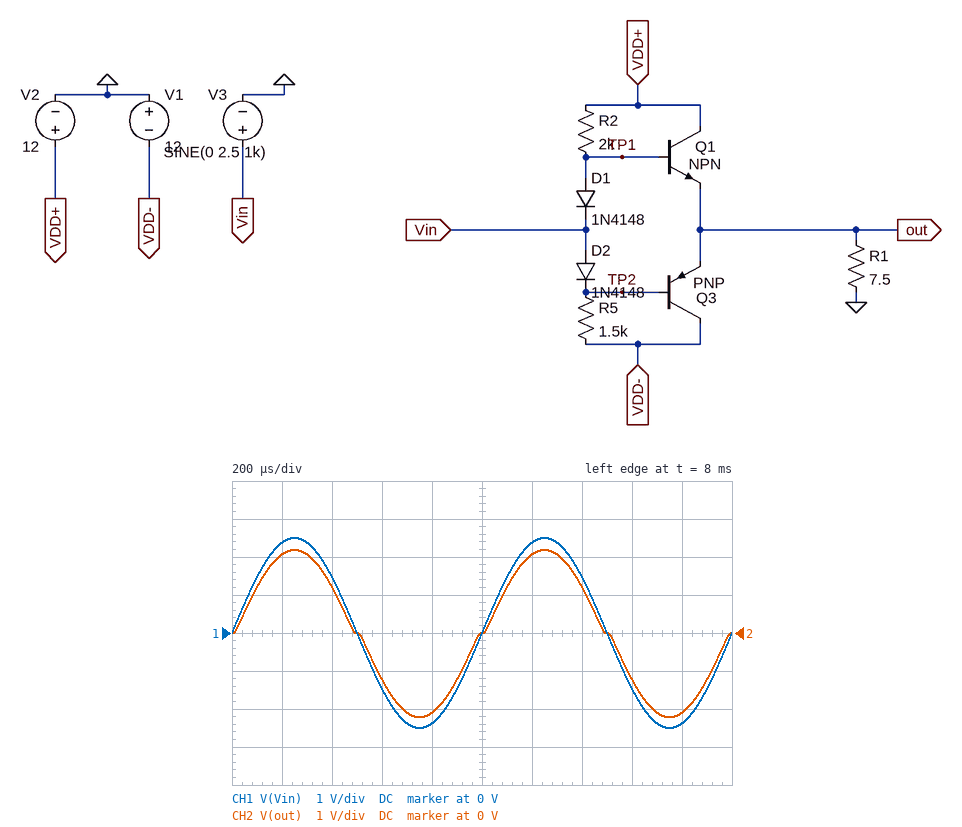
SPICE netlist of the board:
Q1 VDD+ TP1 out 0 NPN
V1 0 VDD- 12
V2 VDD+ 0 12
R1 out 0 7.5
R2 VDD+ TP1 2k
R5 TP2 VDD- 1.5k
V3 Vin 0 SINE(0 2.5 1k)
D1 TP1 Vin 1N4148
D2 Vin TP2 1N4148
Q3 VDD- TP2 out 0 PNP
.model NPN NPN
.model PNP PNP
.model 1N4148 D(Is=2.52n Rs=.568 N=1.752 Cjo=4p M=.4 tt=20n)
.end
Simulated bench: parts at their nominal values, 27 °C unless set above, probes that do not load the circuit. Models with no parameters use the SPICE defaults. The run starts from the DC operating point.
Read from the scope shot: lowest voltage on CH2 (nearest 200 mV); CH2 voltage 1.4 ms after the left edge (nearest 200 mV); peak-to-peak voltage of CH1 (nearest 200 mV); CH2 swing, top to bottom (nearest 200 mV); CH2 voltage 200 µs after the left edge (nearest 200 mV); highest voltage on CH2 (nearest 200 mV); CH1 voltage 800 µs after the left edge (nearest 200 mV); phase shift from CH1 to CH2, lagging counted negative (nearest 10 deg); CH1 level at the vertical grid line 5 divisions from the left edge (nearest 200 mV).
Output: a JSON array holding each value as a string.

["-2.2 V", "1.2 V", "5.0 V", "4.4 V", "2.0 V", "2.2 V", "-2.4 V", "0 deg", "0 V"]
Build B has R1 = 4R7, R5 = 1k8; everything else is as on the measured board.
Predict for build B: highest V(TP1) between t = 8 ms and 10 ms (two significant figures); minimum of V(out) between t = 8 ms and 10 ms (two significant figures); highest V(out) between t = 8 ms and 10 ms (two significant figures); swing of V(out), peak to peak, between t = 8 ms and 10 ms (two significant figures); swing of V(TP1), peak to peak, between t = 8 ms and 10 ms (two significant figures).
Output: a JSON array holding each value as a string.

["3.0 V", "-2.1 V", "2.1 V", "4.2 V", "4.8 V"]
